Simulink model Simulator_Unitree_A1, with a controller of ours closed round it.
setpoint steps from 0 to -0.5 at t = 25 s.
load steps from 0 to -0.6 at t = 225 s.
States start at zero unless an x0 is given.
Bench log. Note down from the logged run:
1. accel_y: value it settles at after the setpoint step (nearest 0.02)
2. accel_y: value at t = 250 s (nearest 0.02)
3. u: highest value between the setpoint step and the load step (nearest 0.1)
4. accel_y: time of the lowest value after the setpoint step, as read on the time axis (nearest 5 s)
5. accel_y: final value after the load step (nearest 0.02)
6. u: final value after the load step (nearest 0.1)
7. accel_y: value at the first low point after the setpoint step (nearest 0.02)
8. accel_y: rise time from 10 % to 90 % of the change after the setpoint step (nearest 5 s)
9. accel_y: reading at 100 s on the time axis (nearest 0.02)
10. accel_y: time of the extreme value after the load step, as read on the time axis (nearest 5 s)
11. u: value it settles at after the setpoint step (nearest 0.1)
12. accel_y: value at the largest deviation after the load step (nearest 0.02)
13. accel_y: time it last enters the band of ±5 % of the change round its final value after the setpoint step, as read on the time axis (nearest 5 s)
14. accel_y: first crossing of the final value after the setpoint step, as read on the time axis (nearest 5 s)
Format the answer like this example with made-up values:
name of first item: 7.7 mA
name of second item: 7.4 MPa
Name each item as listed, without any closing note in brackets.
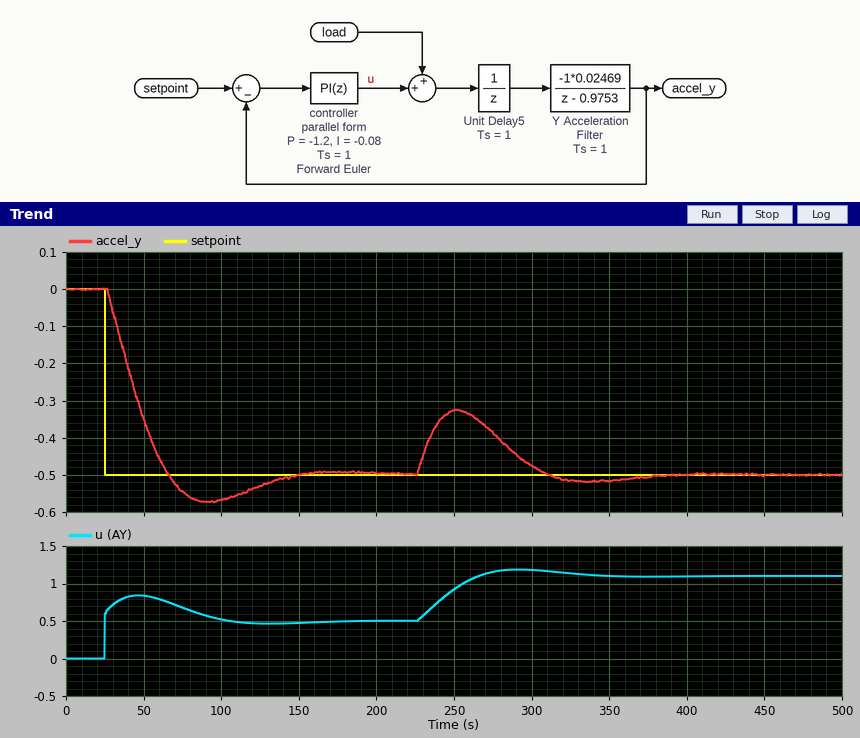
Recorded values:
accel_y: value it settles at after the setpoint step: -0.50
accel_y: value at t = 250 s: -0.32
u: highest value between the setpoint step and the load step: 0.8
accel_y: time of the lowest value after the setpoint step, as read on the time axis: 90 s
accel_y: final value after the load step: -0.50
u: final value after the load step: 1.1
accel_y: value at the first low point after the setpoint step: -0.58
accel_y: rise time from 10 % to 90 % of the change after the setpoint step: 30 s
accel_y: reading at 100 s on the time axis: -0.56
accel_y: time of the extreme value after the load step, as read on the time axis: 250 s
u: value it settles at after the setpoint step: 0.5
accel_y: value at the largest deviation after the load step: -0.32
accel_y: time it last enters the band of ±5 % of the change round its final value after the setpoint step, as read on the time axis: 130 s
accel_y: first crossing of the final value after the setpoint step, as read on the time axis: 65 s
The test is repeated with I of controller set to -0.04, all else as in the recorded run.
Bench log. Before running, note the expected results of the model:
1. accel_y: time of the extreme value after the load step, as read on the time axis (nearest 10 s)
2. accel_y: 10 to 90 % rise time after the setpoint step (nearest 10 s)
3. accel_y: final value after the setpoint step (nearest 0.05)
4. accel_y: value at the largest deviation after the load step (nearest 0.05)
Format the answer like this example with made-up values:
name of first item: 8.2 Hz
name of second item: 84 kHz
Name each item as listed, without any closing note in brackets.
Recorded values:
accel_y: time of the extreme value after the load step, as read on the time axis: 260 s
accel_y: 10 to 90 % rise time after the setpoint step: 50 s
accel_y: final value after the setpoint step: -0.50
accel_y: value at the largest deviation after the load step: -0.30
